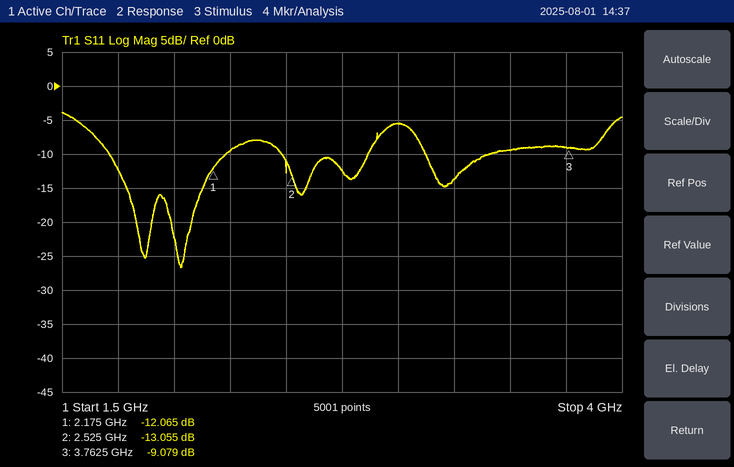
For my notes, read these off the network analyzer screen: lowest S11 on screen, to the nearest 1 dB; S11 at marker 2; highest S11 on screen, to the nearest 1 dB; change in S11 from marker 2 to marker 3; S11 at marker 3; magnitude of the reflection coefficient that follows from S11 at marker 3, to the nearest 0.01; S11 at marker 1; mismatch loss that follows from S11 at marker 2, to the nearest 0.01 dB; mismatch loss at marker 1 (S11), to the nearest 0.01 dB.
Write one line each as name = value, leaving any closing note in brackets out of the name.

lowest S11 on screen, to the nearest 1 dB = -27 dB
S11 at marker 2 = -13.055 dB
highest S11 on screen, to the nearest 1 dB = -4 dB
change in S11 from marker 2 to marker 3 = 3.976 dB
S11 at marker 3 = -9.079 dB
magnitude of the reflection coefficient that follows from S11 at marker 3, to the nearest 0.01 = 0.35
S11 at marker 1 = -12.065 dB
mismatch loss that follows from S11 at marker 2, to the nearest 0.01 dB = 0.22 dB
mismatch loss at marker 1 (S11), to the nearest 0.01 dB = 0.28 dB
